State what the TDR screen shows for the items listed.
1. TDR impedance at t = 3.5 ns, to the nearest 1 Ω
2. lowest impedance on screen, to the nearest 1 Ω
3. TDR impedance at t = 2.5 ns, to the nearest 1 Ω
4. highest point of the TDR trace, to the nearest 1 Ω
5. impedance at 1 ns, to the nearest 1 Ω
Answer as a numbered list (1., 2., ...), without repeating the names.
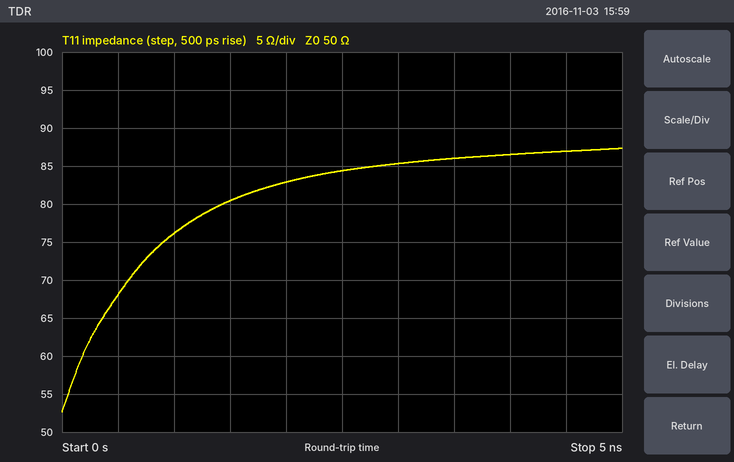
1. 86 Ω
2. 53 Ω
3. 84 Ω
4. 87 Ω
5. 76 Ω
